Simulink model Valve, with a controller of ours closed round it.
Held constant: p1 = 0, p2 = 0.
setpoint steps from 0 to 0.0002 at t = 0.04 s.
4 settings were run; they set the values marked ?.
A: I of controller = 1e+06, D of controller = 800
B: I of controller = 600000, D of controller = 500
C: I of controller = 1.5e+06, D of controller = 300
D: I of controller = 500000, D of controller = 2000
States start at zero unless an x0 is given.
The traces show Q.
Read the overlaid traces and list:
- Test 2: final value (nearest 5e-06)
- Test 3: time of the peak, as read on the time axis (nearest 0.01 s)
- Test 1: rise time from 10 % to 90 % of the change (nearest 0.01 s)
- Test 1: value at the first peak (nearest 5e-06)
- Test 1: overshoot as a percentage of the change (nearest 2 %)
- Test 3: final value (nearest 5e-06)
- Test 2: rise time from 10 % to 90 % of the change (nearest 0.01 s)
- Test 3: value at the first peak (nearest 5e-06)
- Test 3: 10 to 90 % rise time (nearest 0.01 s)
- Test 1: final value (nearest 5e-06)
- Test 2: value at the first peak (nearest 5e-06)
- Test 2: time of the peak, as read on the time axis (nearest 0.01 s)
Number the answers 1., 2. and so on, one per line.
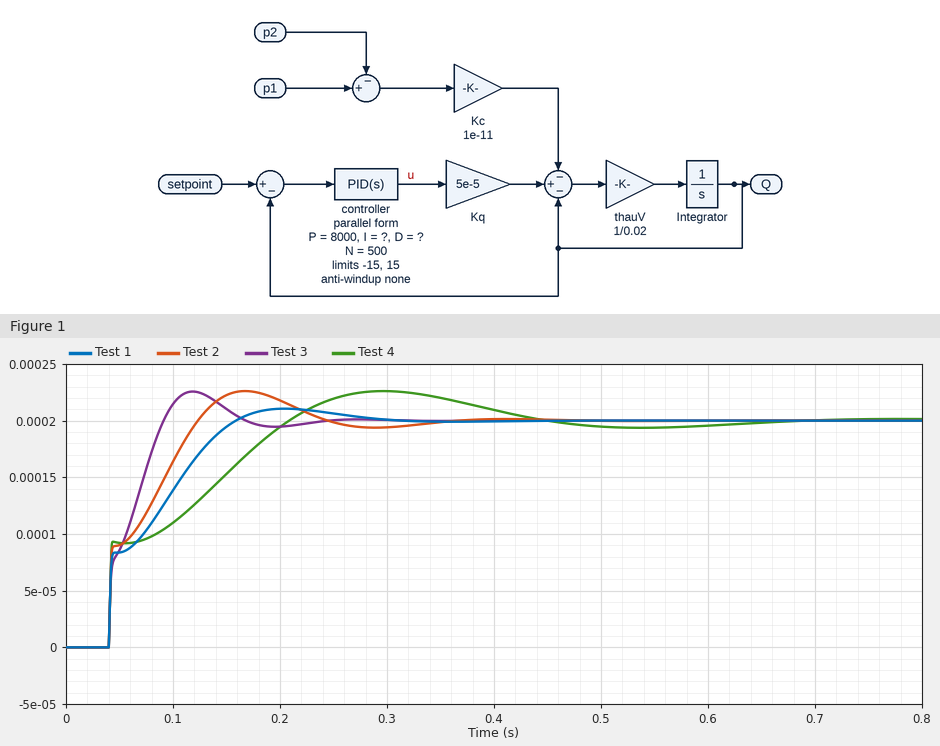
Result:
1. 0.000200
2. 0.12 s
3. 0.09 s
4. 0.000210
5. 6 %
6. 0.000200
7. 0.07 s
8. 0.000225
9. 0.04 s
10. 0.000200
11. 0.000225
12. 0.17 s
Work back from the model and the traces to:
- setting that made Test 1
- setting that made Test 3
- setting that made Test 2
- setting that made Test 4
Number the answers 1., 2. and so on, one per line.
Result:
1. B
2. C
3. A
4. D
